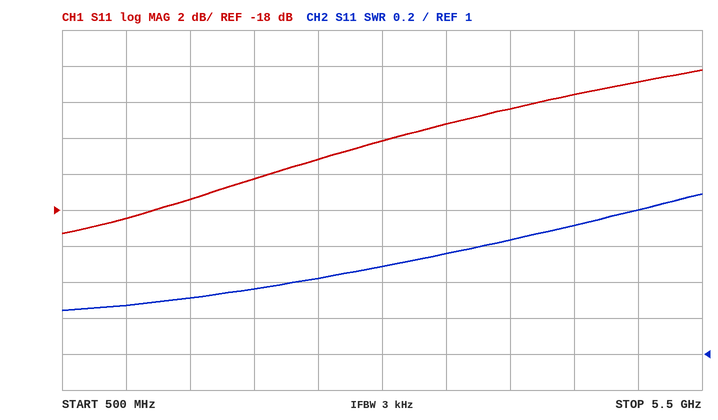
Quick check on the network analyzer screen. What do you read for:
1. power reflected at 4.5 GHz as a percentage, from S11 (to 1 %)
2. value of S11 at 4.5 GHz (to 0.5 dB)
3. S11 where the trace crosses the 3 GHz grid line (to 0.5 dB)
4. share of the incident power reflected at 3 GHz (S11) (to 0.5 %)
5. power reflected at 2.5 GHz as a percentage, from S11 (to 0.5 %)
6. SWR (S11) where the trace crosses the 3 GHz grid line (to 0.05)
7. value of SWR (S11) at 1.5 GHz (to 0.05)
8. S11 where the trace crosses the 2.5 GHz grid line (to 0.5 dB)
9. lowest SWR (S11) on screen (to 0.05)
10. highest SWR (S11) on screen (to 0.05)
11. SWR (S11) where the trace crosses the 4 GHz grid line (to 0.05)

7 %
-11.5 dB
-14.0 dB
4.0 %
3.0 %
1.50
1.30
-15.0 dB
1.25
1.90
1.65
